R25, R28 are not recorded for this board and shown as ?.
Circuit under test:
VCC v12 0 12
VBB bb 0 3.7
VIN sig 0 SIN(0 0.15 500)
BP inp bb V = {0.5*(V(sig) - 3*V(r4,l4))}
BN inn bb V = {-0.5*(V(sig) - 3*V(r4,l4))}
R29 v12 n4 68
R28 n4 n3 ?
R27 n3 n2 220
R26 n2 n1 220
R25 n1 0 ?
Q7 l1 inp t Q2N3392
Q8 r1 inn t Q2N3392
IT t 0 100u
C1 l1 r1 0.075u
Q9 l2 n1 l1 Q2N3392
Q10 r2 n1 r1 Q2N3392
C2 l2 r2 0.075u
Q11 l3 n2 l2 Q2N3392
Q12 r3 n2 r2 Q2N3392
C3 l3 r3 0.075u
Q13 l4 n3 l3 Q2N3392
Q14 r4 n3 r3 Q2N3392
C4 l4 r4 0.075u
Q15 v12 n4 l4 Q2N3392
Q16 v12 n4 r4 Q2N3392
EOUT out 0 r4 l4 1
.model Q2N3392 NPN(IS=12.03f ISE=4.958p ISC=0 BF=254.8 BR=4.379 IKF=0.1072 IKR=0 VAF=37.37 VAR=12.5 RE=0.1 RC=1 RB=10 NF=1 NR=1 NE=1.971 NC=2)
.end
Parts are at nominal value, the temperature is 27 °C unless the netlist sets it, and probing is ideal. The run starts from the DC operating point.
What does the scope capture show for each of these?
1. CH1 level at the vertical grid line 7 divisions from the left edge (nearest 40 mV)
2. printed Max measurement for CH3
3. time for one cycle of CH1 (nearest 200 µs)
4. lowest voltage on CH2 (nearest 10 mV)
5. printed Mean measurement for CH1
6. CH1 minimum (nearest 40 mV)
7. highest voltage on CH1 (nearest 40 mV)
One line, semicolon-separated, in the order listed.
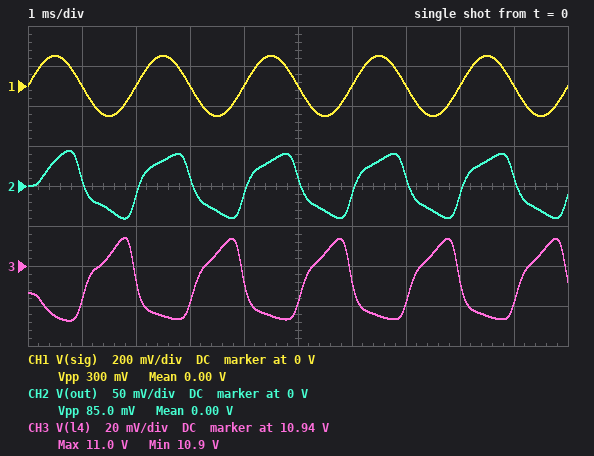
0 V; 11.0 V; 2.0 ms; -40 mV; 0.00 V; -160 mV; 160 mV
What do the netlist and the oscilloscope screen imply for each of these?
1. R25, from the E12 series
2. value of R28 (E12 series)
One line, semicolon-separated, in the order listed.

1 kΩ; 120 Ω
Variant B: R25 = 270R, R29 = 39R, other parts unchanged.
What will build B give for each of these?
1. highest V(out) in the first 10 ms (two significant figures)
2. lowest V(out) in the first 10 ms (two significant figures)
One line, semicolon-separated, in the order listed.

38 mV; -37 mV
